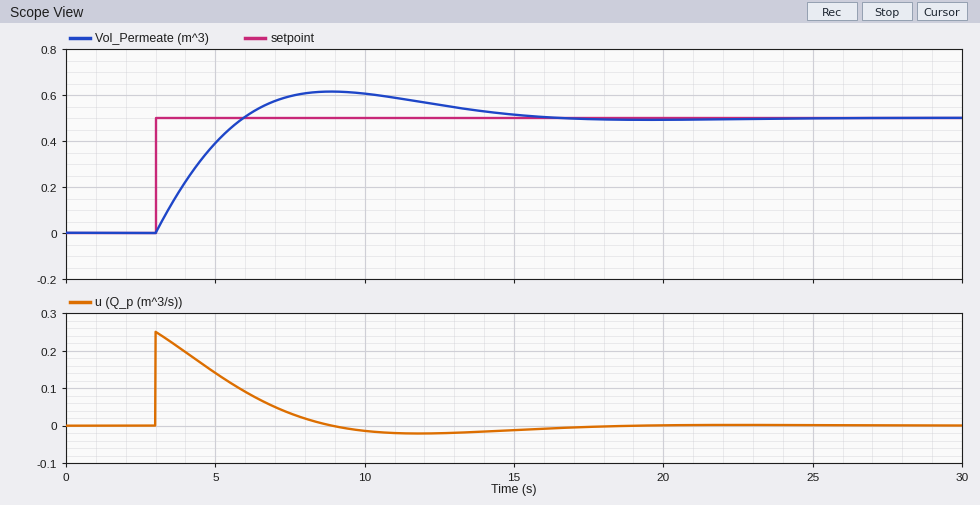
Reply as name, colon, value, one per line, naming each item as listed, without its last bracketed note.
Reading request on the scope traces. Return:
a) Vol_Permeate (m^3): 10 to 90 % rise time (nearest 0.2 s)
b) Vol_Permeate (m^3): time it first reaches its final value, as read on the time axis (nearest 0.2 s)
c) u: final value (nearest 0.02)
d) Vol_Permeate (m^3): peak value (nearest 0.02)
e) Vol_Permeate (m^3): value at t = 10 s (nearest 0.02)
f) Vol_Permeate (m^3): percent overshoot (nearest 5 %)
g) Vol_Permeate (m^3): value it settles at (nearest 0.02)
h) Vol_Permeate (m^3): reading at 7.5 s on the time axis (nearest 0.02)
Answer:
Vol_Permeate (m^3): 10 to 90 % rise time: 2.2 s
Vol_Permeate (m^3): time it first reaches its final value, as read on the time axis: 6.0 s
u: final value: 0.00
Vol_Permeate (m^3): peak value: 0.62
Vol_Permeate (m^3): value at t = 10 s: 0.60
Vol_Permeate (m^3): percent overshoot: 25 %
Vol_Permeate (m^3): value it settles at: 0.50
Vol_Permeate (m^3): reading at 7.5 s on the time axis: 0.60
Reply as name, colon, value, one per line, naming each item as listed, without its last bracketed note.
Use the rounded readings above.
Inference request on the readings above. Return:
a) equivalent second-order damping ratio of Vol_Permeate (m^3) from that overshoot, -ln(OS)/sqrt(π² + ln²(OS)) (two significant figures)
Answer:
equivalent second-order damping ratio of Vol_Permeate (m^3) from that overshoot, -ln(OS)/sqrt(π² + ln²(OS)): 0.40
